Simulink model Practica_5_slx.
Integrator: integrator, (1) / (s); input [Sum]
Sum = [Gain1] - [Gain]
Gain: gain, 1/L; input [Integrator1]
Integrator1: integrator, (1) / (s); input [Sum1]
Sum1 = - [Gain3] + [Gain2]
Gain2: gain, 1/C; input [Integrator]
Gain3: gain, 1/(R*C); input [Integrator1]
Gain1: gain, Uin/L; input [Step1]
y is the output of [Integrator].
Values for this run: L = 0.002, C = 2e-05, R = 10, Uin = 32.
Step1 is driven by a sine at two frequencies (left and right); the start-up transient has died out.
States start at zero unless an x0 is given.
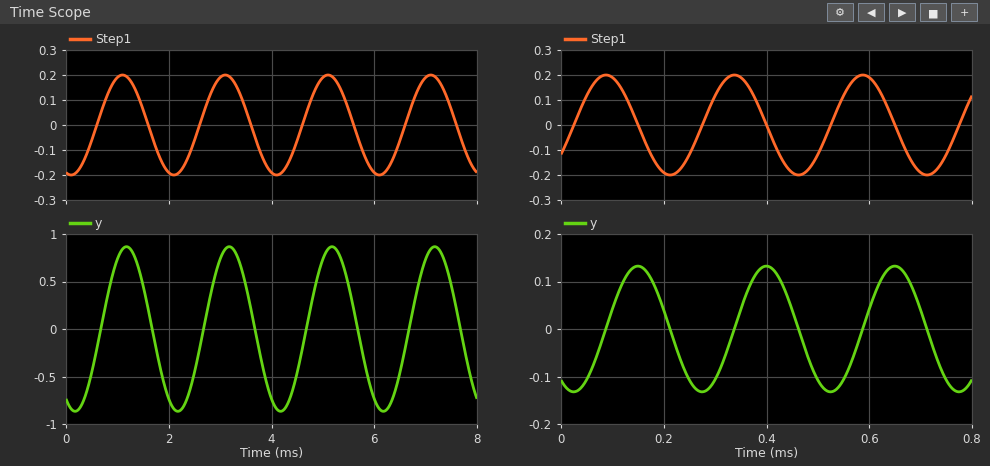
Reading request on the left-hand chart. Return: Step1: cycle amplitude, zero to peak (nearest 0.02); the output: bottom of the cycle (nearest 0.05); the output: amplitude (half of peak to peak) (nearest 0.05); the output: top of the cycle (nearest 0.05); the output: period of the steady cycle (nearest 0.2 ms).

0.20
-0.85
0.85
0.85
2.0 ms
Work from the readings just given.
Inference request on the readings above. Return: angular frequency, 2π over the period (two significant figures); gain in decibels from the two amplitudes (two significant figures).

3.1 rad/ms
13 dB
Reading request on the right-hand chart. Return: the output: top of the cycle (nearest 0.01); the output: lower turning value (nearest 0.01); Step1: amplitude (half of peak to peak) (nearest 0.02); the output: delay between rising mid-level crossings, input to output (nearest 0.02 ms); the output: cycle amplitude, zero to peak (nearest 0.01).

0.13
-0.13
0.20
0.06 ms
0.13
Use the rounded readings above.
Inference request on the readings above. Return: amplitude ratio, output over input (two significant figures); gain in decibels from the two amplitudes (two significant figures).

0.65
-3.7 dB
